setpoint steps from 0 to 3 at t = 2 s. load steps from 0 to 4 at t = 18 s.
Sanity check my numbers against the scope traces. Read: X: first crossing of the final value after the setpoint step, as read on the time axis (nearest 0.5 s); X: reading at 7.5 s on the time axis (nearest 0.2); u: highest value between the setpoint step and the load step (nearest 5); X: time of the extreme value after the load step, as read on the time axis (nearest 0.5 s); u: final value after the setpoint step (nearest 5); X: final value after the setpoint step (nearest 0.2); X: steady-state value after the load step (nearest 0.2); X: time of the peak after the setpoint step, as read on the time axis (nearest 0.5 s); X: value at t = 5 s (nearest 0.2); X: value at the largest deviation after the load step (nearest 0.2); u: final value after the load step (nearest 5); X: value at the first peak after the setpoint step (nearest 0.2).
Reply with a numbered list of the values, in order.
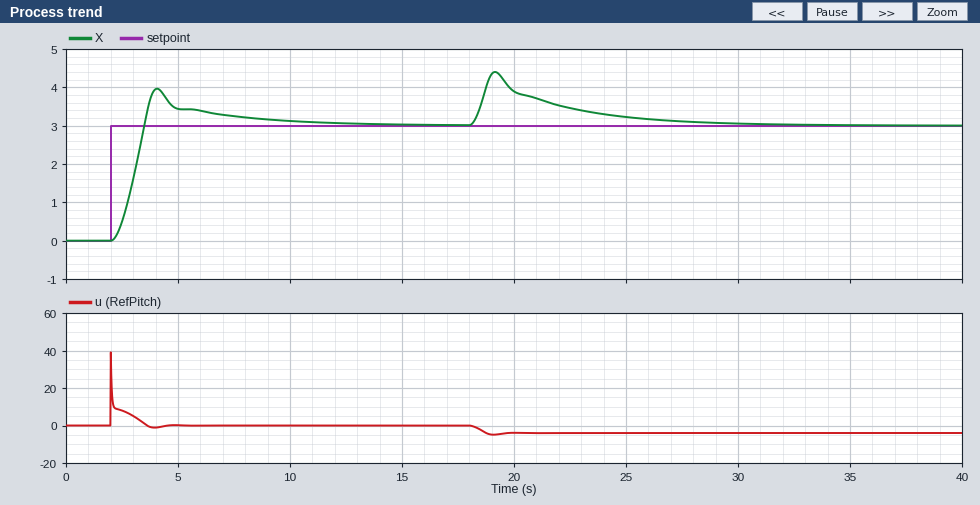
1. 3.5 s
2. 3.2
3. 40
4. 19.0 s
5. 0
6. 3.0
7. 3.0
8. 4.0 s
9. 3.4
10. 4.4
11. -5
12. 4.0
